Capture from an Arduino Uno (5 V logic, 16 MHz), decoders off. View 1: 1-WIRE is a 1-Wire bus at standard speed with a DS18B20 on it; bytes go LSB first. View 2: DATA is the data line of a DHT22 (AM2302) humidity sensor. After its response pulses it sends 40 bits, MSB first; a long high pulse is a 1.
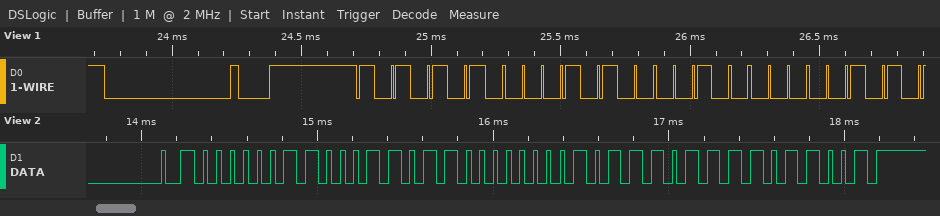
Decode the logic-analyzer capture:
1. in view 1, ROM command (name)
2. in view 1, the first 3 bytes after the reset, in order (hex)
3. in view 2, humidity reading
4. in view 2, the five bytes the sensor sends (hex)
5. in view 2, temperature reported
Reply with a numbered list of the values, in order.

1. Match ROM
2. 55 28 04
3. 79.5 %
4. 03 1B 00 BB D9
5. 18.7 °C
